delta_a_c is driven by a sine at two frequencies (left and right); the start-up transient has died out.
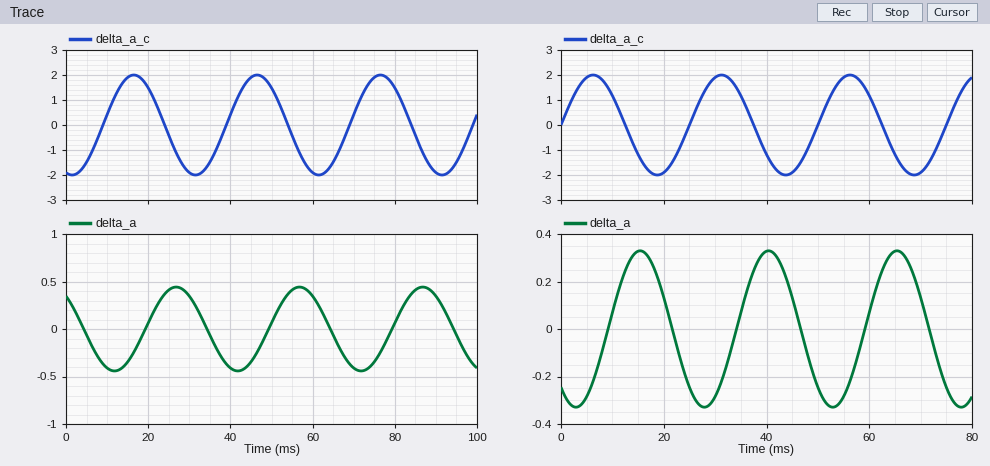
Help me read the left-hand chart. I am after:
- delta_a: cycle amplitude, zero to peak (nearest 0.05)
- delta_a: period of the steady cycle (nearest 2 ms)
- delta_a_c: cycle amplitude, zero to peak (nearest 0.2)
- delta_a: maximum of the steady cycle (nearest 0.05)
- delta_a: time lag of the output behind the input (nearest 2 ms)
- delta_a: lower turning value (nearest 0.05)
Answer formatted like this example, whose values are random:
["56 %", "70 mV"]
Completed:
["0.45", "30 ms", "2.0", "0.45", "10 ms", "-0.45"]
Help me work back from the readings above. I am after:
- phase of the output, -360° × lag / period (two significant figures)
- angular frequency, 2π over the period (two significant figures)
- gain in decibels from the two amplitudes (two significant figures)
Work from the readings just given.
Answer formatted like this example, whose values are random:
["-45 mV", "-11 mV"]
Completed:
["-120°", "0.21 rad/ms", "-13 dB"]
